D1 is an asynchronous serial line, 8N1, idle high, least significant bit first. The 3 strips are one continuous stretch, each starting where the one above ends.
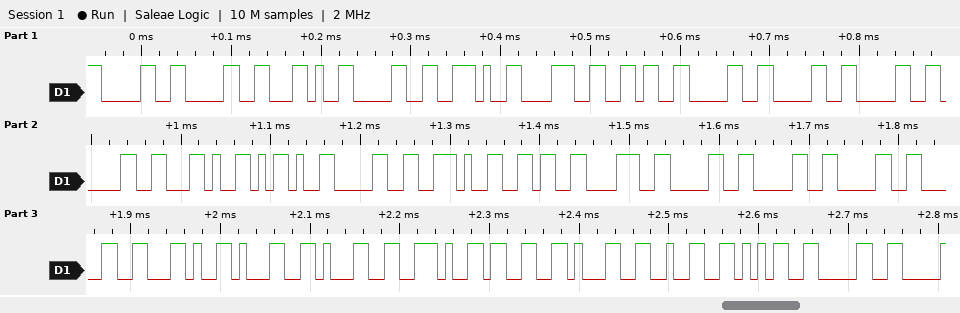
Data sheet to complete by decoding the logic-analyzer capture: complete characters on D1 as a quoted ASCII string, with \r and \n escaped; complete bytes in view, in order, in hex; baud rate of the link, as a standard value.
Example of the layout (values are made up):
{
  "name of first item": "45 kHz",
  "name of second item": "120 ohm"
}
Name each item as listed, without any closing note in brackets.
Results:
{
  "complete characters on D1 as a quoted ASCII string, with \\r and \\n escaped": "\"00,0.860000,-0.680000,11.31250\"",
  "complete bytes in view, in order, in hex": "30 30 2C 30 2E 38 36 30 30 30 30 2C 2D 30 2E 36 38 30 30 30 30 2C 31 31 2E 33 31 32 35 30",
  "baud rate of the link, as a standard value": "115200 baud"
}
